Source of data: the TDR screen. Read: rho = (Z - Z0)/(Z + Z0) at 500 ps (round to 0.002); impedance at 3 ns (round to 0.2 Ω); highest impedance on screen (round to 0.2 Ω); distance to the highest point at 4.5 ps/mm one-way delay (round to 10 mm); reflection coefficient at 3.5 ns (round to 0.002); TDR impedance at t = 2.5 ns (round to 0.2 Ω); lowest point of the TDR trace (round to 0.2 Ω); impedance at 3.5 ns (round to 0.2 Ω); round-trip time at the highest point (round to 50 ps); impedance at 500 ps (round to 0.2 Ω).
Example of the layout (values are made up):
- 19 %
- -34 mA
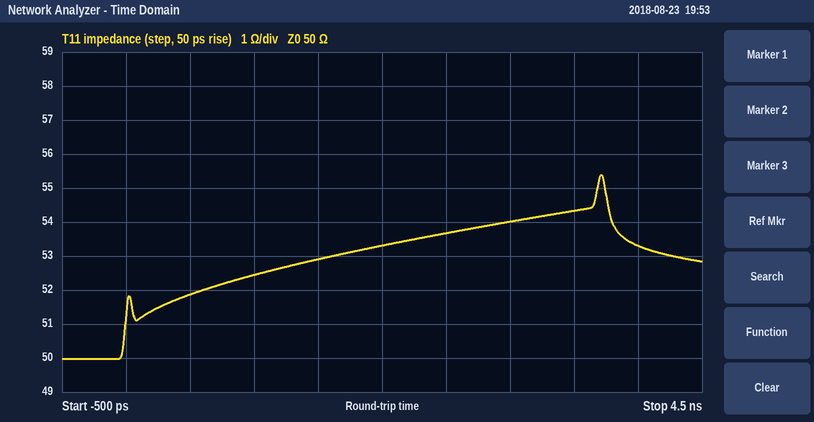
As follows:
- +0.018
- 54.0 Ω
- 55.4 Ω
- 410 mm
- +0.042
- 53.6 Ω
- 50.0 Ω
- 54.4 Ω
- 3.70 ns
- 51.8 Ω
